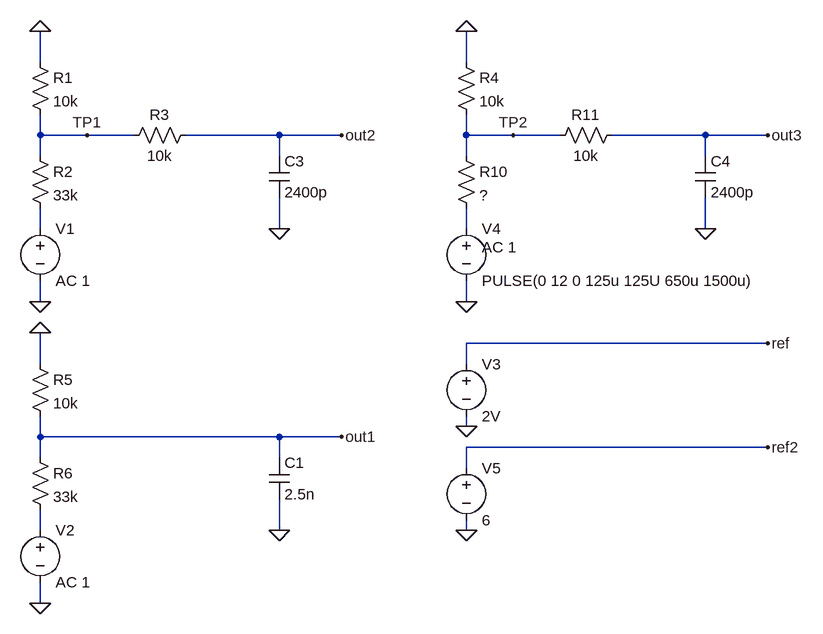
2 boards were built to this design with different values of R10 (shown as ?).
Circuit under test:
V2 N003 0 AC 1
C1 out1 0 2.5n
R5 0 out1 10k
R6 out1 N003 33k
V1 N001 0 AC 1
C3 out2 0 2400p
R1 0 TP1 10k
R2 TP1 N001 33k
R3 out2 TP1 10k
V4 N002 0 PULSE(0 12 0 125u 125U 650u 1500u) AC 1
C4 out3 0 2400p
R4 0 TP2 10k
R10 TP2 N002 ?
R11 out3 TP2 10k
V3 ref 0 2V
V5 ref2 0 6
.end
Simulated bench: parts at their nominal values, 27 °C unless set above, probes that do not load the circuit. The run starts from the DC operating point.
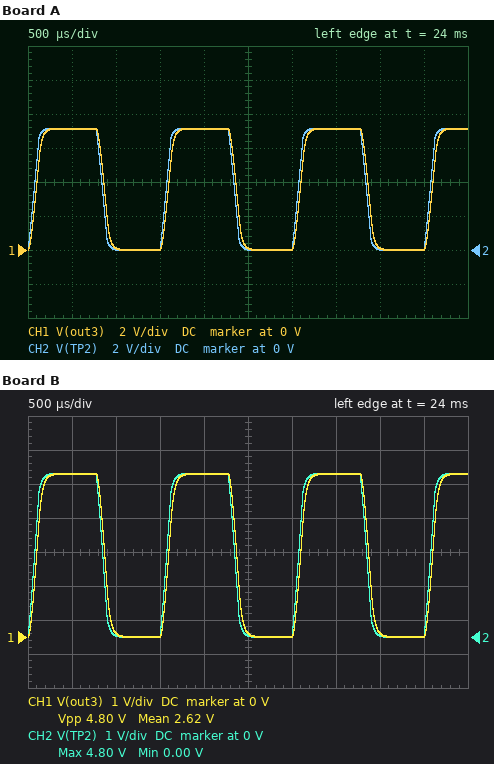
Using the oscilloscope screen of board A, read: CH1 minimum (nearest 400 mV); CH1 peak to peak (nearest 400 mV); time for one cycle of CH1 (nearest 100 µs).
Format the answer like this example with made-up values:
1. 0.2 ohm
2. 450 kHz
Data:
1. 0 V
2. 7.2 V
3. 1.5 ms
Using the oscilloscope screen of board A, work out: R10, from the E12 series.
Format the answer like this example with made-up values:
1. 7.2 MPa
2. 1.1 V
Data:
1. 6.8 kΩ
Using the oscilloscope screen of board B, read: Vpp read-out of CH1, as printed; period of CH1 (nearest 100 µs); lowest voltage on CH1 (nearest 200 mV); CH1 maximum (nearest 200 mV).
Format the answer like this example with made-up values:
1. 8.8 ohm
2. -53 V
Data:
1. 4.80 V
2. 1.5 ms
3. 0 V
4. 4.8 V
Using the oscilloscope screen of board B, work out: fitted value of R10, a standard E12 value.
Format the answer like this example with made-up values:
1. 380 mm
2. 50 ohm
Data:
1. 15 kΩ
